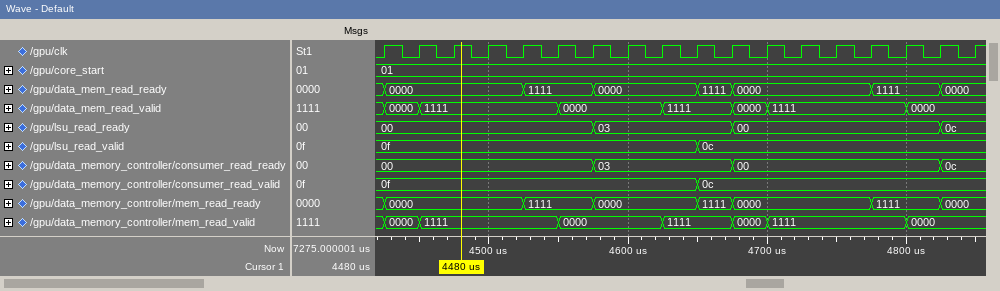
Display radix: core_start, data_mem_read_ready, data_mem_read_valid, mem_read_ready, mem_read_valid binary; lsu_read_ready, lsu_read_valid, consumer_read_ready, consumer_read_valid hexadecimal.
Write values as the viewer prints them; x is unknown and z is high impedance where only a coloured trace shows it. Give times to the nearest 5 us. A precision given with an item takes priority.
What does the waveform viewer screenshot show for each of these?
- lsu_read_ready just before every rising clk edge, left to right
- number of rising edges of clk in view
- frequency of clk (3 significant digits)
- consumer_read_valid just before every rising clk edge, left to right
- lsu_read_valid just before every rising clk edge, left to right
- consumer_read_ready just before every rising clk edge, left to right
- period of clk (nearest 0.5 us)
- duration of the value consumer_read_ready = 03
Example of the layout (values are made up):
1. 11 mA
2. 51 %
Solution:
1. 00, 00, 00, 00, 00, 00, 00, 03, 03, 03, 03, 00, 00, 00, 00, 00, 00, 0c
2. 18
3. 40.0 kHz
4. 0f, 0f, 0f, 0f, 0f, 0f, 0f, 0f, 0f, 0f, 0c, 0c, 0c, 0c, 0c, 0c, 0c, 0c
5. 0f, 0f, 0f, 0f, 0f, 0f, 0f, 0f, 0f, 0f, 0c, 0c, 0c, 0c, 0c, 0c, 0c, 0c
6. 00, 00, 00, 00, 00, 00, 00, 03, 03, 03, 03, 00, 00, 00, 00, 00, 00, 0c
7. 25 us
8. 100 us
